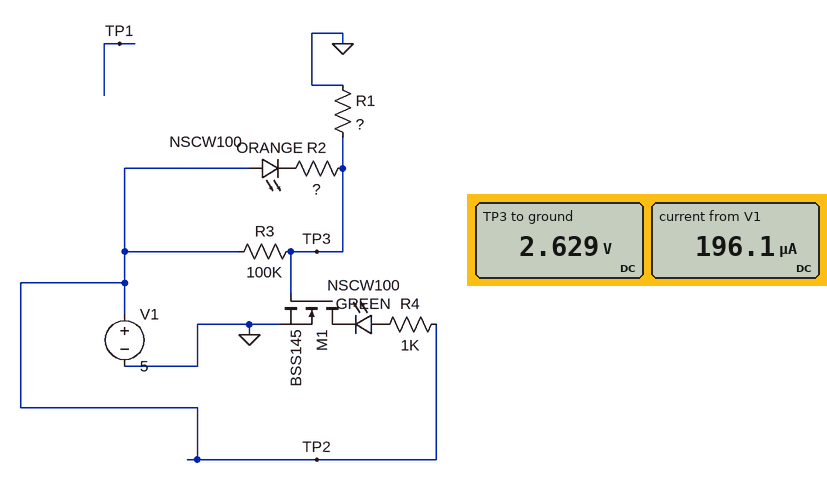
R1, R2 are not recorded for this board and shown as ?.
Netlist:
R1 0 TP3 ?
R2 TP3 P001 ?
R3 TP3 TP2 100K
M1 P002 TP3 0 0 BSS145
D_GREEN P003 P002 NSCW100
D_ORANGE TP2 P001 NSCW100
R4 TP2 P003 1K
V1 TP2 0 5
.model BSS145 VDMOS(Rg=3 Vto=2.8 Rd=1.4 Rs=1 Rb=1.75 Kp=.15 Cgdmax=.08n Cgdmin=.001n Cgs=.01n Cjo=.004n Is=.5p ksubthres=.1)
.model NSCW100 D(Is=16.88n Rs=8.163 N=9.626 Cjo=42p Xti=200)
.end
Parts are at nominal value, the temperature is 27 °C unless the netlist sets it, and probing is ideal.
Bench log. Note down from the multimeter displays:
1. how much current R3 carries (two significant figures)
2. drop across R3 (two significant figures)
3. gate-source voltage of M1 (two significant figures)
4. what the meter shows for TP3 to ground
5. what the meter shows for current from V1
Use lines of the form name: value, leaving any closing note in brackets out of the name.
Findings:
how much current R3 carries: 24 µA
drop across R3: 2.4 V
gate-source voltage of M1: 2.6 V
what the meter shows for TP3 to ground: 2.629 V
what the meter shows for current from V1: 196.1 µA
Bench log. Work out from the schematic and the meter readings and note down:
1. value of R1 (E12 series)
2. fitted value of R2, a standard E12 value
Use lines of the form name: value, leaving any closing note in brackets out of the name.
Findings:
value of R1: 15 kΩ
fitted value of R2, a standard E12 value: 680 Ω
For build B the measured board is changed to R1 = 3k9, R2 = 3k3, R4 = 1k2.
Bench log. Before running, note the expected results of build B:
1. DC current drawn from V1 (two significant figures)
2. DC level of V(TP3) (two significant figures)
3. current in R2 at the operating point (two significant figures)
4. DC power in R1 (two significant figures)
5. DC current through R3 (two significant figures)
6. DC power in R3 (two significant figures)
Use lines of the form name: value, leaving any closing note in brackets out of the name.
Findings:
DC current drawn from V1: 370 µA
DC level of V(TP3): 1.4 V
current in R2 at the operating point: 330 µA
DC power in R1: 530 µW
DC current through R3: 36 µA
DC power in R3: 130 µW
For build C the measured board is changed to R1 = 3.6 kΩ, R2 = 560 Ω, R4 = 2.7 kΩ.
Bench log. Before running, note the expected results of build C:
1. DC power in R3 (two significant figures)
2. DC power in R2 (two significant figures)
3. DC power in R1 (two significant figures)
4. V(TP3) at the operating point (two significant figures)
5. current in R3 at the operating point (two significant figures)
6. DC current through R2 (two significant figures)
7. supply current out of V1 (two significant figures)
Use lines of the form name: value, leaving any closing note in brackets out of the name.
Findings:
DC power in R3: 84 µW
DC power in R2: 170 µW
DC power in R1: 1.2 mW
V(TP3) at the operating point: 2.1 V
current in R3 at the operating point: 29 µA
DC current through R2: 550 µA
supply current out of V1: 580 µA
